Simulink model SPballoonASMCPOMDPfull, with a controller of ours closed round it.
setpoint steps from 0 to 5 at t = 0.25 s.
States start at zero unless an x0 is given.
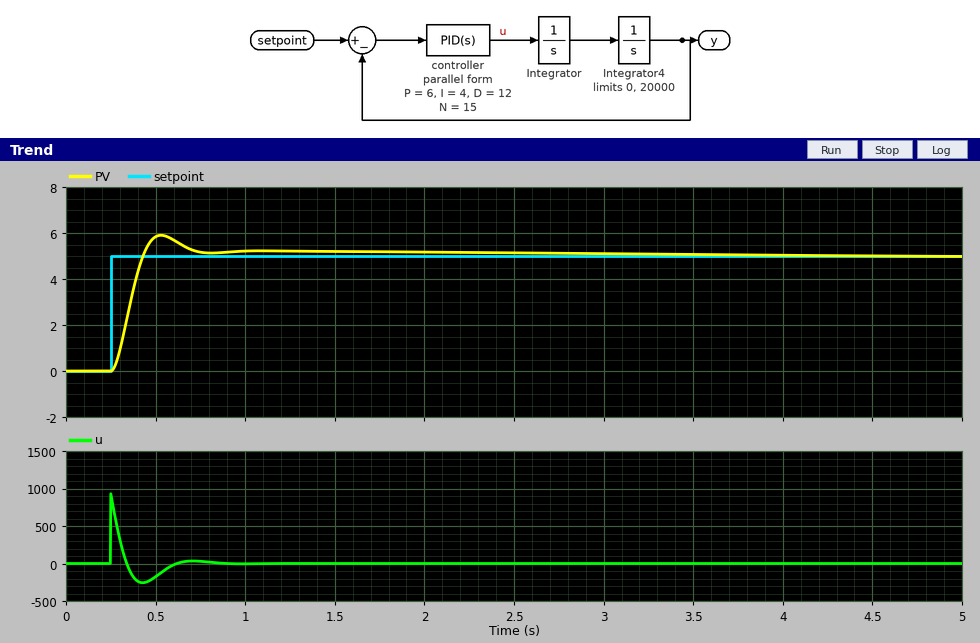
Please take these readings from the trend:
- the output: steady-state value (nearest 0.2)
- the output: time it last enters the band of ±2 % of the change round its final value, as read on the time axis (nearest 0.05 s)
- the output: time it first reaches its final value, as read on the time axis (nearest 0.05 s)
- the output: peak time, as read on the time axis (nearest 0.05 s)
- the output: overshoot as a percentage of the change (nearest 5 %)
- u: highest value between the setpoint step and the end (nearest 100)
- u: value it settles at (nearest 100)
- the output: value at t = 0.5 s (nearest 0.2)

5.0
3.00 s
0.45 s
0.55 s
20 %
900
0
5.8
